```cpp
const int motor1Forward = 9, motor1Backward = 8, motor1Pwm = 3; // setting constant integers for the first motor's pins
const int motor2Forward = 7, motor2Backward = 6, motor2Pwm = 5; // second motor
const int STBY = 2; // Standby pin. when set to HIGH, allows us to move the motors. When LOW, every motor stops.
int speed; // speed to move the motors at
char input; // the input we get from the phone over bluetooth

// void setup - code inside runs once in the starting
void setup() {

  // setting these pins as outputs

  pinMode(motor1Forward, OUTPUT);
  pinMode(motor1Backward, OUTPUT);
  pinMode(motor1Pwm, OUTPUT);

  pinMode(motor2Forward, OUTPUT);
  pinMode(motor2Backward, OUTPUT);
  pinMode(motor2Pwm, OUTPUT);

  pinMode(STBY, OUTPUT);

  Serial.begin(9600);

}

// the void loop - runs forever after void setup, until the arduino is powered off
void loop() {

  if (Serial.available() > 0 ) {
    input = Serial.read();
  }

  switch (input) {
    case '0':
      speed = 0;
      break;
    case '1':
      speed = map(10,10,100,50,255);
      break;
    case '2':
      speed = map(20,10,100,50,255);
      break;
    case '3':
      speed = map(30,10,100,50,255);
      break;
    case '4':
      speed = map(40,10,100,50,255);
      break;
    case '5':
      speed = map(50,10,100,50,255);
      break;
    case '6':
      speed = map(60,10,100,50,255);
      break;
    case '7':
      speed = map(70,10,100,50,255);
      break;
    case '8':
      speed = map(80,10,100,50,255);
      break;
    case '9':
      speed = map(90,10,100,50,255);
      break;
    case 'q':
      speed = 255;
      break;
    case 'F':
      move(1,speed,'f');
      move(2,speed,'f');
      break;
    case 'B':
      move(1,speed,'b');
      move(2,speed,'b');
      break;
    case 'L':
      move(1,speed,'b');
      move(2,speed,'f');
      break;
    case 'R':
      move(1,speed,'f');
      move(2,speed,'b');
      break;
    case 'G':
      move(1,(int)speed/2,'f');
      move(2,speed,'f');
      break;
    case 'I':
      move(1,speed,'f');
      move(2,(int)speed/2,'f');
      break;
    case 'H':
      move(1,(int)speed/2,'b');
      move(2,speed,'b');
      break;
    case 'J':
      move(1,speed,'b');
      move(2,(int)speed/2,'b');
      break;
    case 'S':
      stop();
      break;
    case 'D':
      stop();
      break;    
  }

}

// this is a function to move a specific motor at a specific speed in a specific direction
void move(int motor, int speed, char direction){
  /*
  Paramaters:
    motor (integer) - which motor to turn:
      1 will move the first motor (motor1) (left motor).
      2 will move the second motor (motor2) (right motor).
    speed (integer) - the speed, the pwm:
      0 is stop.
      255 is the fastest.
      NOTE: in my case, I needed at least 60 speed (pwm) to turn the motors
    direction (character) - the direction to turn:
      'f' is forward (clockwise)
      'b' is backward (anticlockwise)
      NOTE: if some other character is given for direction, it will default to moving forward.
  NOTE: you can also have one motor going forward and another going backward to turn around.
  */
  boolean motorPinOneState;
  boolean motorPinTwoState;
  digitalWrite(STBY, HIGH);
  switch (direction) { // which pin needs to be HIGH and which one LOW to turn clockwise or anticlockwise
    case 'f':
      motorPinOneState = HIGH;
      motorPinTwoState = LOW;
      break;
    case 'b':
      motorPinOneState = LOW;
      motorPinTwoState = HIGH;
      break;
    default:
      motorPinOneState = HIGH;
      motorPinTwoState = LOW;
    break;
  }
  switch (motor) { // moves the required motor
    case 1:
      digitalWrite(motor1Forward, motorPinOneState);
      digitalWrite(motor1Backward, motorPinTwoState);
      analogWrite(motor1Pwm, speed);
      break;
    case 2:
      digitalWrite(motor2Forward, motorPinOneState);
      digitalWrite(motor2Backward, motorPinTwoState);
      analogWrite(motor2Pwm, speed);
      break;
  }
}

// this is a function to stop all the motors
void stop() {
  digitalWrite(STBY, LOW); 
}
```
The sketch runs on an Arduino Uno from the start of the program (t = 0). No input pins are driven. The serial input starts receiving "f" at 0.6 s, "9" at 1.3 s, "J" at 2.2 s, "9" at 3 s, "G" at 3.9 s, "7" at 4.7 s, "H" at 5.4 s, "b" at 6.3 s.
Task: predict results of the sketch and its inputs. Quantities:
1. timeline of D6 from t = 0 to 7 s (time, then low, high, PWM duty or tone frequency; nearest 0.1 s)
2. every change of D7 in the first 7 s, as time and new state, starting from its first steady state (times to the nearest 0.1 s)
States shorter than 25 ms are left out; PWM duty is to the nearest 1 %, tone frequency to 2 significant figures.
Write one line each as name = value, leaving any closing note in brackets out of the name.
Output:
timeline of D6 from t = 0 to 7 s = 0 s low; 2.2 s high; 3.9 s low; 5.4 s high
every change of D7 in the first 7 s, as time and new state, starting from its first steady state = 0 s low; 3.9 s high; 5.4 s low
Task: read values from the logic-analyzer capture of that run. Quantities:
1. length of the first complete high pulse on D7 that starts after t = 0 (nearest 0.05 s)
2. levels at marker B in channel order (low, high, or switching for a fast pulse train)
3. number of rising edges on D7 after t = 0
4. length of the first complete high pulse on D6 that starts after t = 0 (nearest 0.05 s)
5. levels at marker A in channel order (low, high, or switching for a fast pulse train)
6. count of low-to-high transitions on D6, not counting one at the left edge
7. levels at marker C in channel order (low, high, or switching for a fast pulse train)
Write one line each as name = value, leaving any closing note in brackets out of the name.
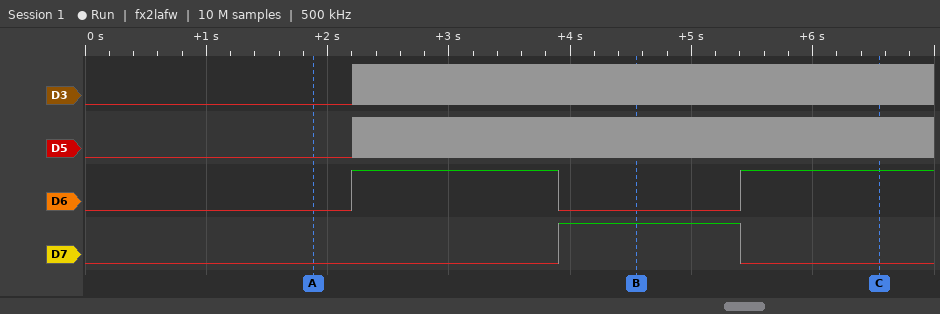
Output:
length of the first complete high pulse on D7 that starts after t = 0 = 1.50 s
levels at marker B in channel order = D3 switching, D5 switching, D6 low, D7 high
number of rising edges on D7 after t = 0 = 1
length of the first complete high pulse on D6 that starts after t = 0 = 1.70 s
levels at marker A in channel order = D3 low, D5 low, D6 low, D7 low
count of low-to-high transitions on D6, not counting one at the left edge = 2
levels at marker C in channel order = D3 switching, D5 switching, D6 high, D7 low
